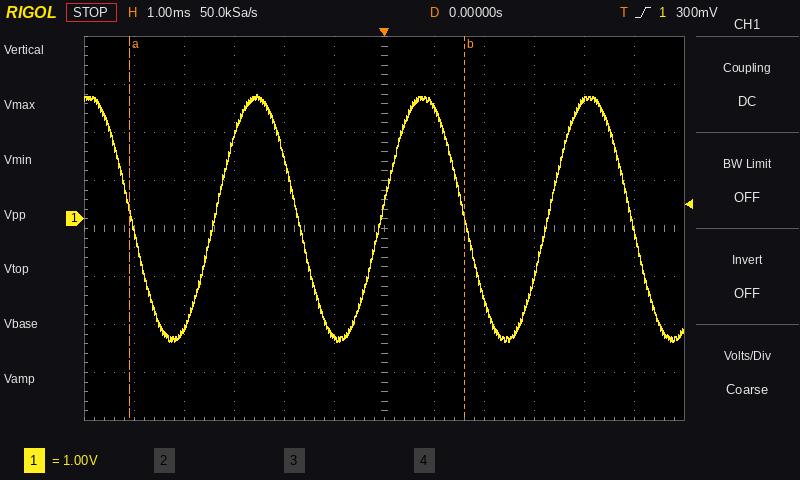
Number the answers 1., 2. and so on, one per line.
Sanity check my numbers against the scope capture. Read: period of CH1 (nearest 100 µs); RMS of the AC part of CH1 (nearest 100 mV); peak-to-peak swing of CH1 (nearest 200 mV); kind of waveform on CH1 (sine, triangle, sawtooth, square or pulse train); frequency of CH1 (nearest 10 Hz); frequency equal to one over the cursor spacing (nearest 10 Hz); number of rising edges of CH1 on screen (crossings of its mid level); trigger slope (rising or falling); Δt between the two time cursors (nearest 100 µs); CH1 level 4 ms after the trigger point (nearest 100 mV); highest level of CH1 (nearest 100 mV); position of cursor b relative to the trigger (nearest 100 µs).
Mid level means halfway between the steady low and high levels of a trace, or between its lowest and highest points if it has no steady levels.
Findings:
1. 3.3 ms
2. 1.8 V
3. 5.2 V
4. sine
5. 300 Hz
6. 150 Hz
7. 3
8. rising
9. 6.7 ms
10. 2.5 V
11. 2.6 V
12. +1.6 ms
